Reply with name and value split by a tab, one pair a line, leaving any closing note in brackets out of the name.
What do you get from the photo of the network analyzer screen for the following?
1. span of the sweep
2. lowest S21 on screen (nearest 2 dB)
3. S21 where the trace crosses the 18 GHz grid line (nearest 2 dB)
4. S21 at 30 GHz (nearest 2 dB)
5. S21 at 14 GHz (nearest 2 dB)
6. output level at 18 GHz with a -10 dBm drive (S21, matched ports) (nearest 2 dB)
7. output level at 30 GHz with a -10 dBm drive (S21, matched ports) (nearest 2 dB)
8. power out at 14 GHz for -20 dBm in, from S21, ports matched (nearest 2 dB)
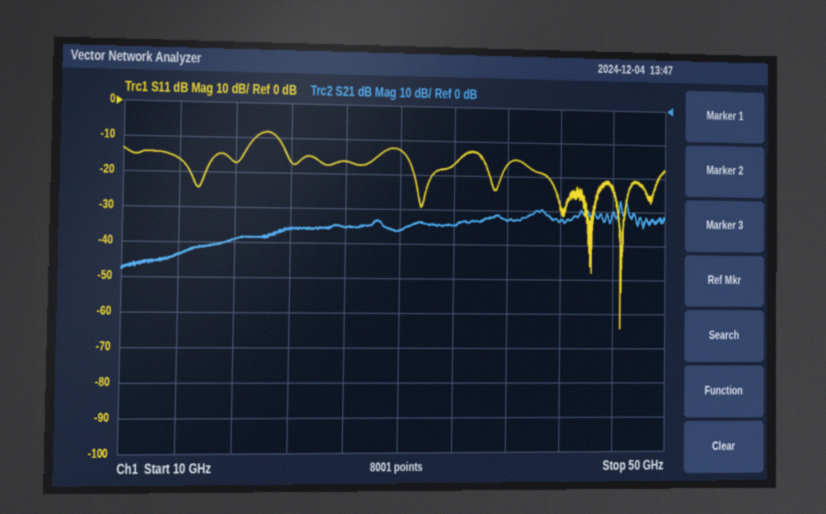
span of the sweep	40 GHz
lowest S21 on screen	-48 dB
S21 where the trace crosses the 18 GHz grid line	-40 dB
S21 at 30 GHz	-36 dB
S21 at 14 GHz	-44 dB
output level at 18 GHz with a -10 dBm drive (S21, matched ports)	-50 dBm
output level at 30 GHz with a -10 dBm drive (S21, matched ports)	-46 dBm
power out at 14 GHz for -20 dBm in, from S21, ports matched	-64 dBm
